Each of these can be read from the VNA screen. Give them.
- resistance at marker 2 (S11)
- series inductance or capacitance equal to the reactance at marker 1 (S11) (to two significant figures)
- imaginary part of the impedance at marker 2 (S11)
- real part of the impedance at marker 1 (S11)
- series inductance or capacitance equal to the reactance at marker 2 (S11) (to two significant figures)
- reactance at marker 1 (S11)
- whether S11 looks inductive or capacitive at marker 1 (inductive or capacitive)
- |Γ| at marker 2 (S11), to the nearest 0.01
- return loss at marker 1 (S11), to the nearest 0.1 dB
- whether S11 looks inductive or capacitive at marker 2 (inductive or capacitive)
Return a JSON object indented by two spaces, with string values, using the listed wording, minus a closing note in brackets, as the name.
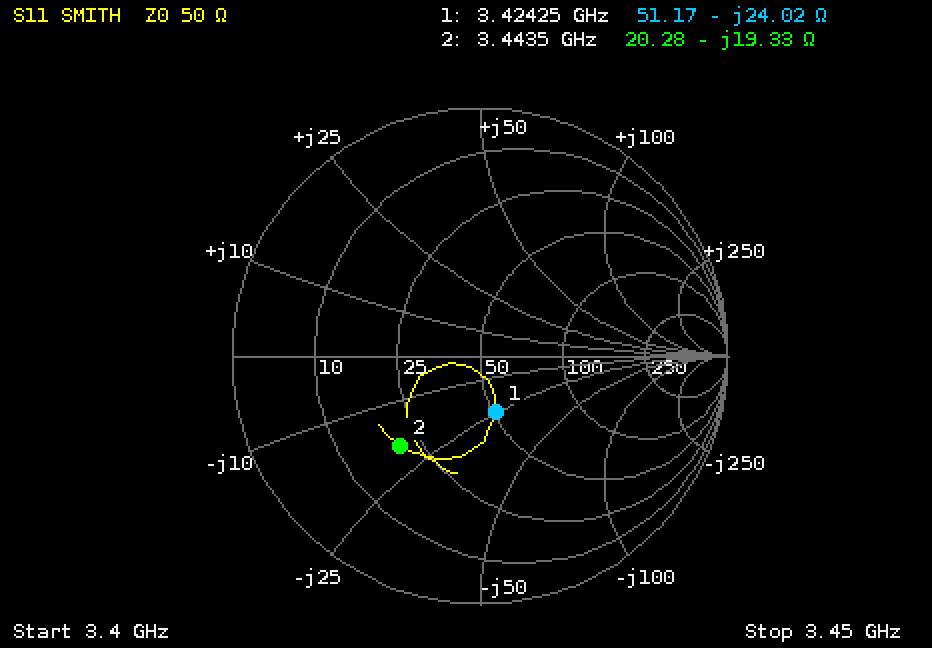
{
  "resistance at marker 2": "20.28 Ω",
  "series inductance or capacitance equal to the reactance at marker 1 (S11)": "1.9 pF",
  "imaginary part of the impedance at marker 2": "-19.33 Ω",
  "real part of the impedance at marker 1": "51.17 Ω",
  "series inductance or capacitance equal to the reactance at marker 2 (S11)": "2.4 pF",
  "reactance at marker 1": "-24.02 Ω",
  "whether S11 looks inductive or capacitive at marker 1": "capacitive",
  "|Γ| at marker 2 (S11), to the nearest 0.01": "0.49",
  "return loss at marker 1 (S11), to the nearest 0.1 dB": "12.7 dB",
  "whether S11 looks inductive or capacitive at marker 2": "capacitive"
}
